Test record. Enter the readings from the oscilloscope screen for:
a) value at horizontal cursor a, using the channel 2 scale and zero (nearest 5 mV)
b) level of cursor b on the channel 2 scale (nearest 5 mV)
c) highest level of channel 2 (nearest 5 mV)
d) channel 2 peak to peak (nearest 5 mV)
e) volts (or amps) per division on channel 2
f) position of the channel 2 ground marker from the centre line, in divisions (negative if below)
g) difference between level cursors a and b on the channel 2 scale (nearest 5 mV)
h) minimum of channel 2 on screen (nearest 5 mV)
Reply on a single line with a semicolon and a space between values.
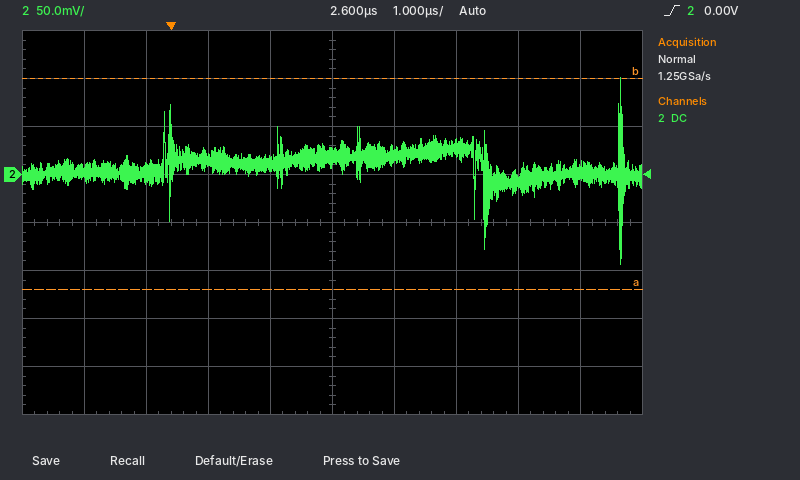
-120 mV; 100 mV; 100 mV; 195 mV; 50 mV; +1.0 div; 220 mV; -95 mV
